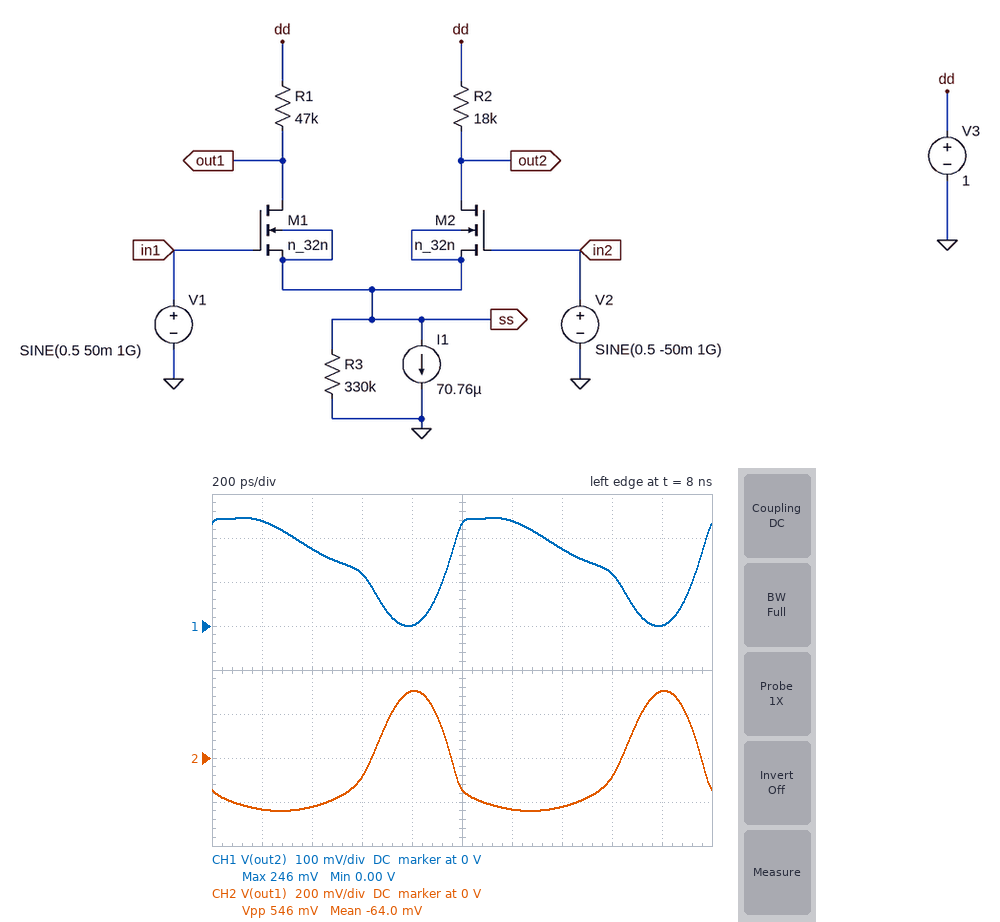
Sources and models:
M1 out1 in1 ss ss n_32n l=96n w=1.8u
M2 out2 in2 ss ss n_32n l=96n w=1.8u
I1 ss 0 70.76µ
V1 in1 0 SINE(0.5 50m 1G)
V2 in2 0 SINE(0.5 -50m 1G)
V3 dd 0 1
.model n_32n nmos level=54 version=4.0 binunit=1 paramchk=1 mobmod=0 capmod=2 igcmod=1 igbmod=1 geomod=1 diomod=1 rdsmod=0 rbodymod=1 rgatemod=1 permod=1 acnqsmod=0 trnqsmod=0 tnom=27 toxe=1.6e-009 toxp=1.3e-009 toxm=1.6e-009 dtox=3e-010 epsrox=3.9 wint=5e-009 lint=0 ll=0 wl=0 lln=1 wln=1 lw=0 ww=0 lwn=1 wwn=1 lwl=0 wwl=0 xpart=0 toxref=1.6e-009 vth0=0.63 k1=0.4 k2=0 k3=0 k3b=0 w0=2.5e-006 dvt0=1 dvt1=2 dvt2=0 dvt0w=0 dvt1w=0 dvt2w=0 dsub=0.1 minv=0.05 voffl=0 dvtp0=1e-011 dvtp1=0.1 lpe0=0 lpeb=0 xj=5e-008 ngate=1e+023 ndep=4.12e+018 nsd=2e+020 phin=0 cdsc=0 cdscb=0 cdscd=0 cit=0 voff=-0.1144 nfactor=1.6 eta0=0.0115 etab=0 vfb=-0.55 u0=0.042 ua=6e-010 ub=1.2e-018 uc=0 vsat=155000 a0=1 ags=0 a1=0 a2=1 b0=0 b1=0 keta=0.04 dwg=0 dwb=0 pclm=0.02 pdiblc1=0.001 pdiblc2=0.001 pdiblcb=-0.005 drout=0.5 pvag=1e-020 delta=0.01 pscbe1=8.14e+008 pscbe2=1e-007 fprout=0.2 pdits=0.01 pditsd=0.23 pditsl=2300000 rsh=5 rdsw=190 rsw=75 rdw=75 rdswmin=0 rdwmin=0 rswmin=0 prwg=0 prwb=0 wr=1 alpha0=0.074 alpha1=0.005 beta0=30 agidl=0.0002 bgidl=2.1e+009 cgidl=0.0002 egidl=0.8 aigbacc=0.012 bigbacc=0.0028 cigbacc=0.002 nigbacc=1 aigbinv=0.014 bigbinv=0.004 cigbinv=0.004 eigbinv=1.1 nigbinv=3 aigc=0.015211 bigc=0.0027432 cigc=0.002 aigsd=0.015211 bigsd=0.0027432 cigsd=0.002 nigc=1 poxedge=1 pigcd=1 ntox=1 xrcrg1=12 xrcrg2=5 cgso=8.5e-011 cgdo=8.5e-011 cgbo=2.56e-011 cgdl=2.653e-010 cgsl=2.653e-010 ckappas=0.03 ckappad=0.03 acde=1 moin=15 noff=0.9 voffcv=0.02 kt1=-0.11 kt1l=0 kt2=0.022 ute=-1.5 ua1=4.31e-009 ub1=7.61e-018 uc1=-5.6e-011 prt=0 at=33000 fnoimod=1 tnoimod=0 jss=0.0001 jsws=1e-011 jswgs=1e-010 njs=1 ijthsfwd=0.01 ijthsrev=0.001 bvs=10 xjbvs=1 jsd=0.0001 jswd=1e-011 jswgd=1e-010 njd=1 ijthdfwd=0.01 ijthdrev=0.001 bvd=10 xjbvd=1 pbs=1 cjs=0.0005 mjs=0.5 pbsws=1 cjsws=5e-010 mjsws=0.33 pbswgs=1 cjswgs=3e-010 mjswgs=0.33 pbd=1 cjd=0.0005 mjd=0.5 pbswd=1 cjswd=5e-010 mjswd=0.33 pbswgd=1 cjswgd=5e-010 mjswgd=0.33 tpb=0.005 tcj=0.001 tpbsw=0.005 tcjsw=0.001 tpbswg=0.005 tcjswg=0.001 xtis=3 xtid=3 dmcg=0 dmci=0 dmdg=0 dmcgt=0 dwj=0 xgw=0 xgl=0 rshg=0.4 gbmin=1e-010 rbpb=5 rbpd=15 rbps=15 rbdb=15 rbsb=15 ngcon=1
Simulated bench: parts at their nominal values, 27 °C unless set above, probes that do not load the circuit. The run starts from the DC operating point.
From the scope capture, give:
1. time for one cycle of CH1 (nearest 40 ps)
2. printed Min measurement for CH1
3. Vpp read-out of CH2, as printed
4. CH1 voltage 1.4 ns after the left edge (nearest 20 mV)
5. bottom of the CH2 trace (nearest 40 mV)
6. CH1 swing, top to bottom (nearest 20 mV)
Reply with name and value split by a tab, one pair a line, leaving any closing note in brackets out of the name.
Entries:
time for one cycle of CH1	1.00 ns
printed Min measurement for CH1	0.00 V
Vpp read-out of CH2, as printed	546 mV
CH1 voltage 1.4 ns after the left edge	180 mV
bottom of the CH2 trace	-240 mV
CH1 swing, top to bottom	240 mV
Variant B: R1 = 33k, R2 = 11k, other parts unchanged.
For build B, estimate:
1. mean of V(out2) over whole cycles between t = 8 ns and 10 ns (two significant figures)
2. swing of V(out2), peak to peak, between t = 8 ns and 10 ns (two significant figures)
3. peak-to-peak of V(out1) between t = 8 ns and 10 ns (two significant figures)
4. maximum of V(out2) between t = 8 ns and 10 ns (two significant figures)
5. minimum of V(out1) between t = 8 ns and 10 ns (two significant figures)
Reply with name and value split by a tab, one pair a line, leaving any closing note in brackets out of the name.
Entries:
mean of V(out2) over whole cycles between t = 8 ns and 10 ns	530 mV
swing of V(out2), peak to peak, between t = 8 ns and 10 ns	270 mV
peak-to-peak of V(out1) between t = 8 ns and 10 ns	750 mV
maximum of V(out2) between t = 8 ns and 10 ns	640 mV
minimum of V(out1) between t = 8 ns and 10 ns	-200 mV
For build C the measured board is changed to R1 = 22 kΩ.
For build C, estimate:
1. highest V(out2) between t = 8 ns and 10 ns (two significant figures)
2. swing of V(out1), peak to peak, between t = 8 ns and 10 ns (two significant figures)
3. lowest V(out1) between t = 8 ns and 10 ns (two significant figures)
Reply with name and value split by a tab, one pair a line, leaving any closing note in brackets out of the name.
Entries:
highest V(out2) between t = 8 ns and 10 ns	660 mV
swing of V(out1), peak to peak, between t = 8 ns and 10 ns	790 mV
lowest V(out1) between t = 8 ns and 10 ns	-120 mV
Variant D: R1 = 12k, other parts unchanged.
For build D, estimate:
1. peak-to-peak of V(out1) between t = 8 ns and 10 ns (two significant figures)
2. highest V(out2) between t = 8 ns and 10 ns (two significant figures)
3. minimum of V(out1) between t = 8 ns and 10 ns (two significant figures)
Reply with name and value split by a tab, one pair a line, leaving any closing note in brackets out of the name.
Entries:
peak-to-peak of V(out1) between t = 8 ns and 10 ns	500 mV
highest V(out2) between t = 8 ns and 10 ns	750 mV
minimum of V(out1) between t = 8 ns and 10 ns	320 mV
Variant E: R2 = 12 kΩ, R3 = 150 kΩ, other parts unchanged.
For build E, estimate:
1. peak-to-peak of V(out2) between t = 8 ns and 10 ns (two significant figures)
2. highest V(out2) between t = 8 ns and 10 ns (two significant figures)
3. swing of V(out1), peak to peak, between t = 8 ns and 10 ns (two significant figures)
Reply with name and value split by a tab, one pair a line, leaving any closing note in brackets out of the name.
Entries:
peak-to-peak of V(out2) between t = 8 ns and 10 ns	180 mV
highest V(out2) between t = 8 ns and 10 ns	510 mV
swing of V(out1), peak to peak, between t = 8 ns and 10 ns	590 mV
